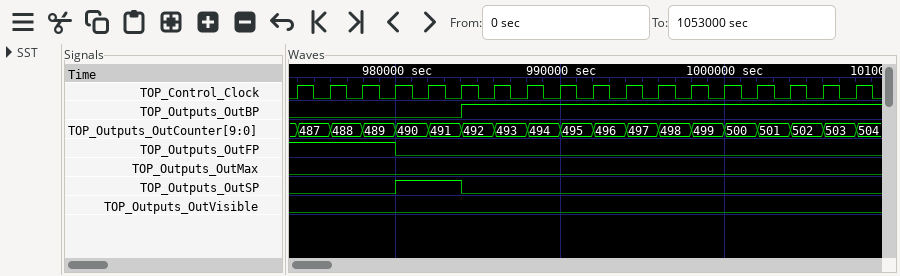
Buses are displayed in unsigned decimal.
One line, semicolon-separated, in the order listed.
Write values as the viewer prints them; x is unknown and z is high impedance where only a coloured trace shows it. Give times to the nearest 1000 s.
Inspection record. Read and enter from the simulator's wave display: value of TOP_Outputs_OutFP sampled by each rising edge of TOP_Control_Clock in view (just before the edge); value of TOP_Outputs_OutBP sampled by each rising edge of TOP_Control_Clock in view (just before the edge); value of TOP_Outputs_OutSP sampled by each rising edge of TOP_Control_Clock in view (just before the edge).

1 1 1 1 0 0 0 0 0 0 0 0 0 0 0 0 0 0; 0 0 0 0 0 0 1 1 1 1 1 1 1 1 1 1 1 1; 0 0 0 0 1 1 0 0 0 0 0 0 0 0 0 0 0 0
